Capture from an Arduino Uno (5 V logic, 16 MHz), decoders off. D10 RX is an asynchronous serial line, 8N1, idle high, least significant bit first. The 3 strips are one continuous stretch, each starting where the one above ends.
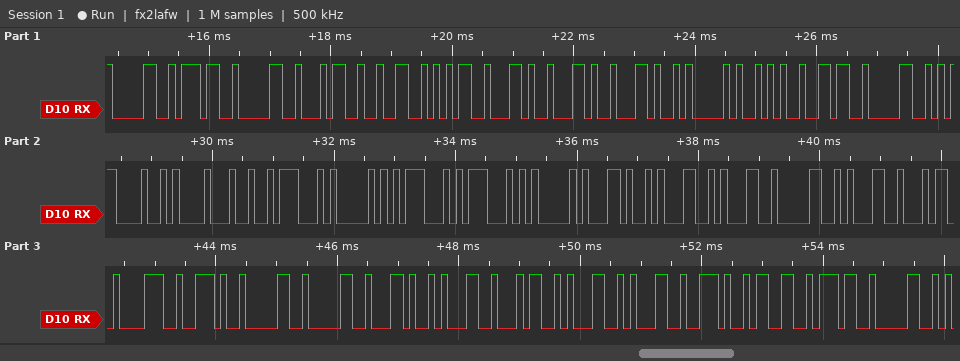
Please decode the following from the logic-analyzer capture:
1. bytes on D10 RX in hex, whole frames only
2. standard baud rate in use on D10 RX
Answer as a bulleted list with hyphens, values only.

- 30 37 30 34 32 35 2C 2C 2C 41 2A 36 30 0D 0A 24 47 50 47 47 41 2C 31 31 30 31 34 38 2E 30 30 2C 31 34 31 31 2E 33 37 30
- 9600 baud
